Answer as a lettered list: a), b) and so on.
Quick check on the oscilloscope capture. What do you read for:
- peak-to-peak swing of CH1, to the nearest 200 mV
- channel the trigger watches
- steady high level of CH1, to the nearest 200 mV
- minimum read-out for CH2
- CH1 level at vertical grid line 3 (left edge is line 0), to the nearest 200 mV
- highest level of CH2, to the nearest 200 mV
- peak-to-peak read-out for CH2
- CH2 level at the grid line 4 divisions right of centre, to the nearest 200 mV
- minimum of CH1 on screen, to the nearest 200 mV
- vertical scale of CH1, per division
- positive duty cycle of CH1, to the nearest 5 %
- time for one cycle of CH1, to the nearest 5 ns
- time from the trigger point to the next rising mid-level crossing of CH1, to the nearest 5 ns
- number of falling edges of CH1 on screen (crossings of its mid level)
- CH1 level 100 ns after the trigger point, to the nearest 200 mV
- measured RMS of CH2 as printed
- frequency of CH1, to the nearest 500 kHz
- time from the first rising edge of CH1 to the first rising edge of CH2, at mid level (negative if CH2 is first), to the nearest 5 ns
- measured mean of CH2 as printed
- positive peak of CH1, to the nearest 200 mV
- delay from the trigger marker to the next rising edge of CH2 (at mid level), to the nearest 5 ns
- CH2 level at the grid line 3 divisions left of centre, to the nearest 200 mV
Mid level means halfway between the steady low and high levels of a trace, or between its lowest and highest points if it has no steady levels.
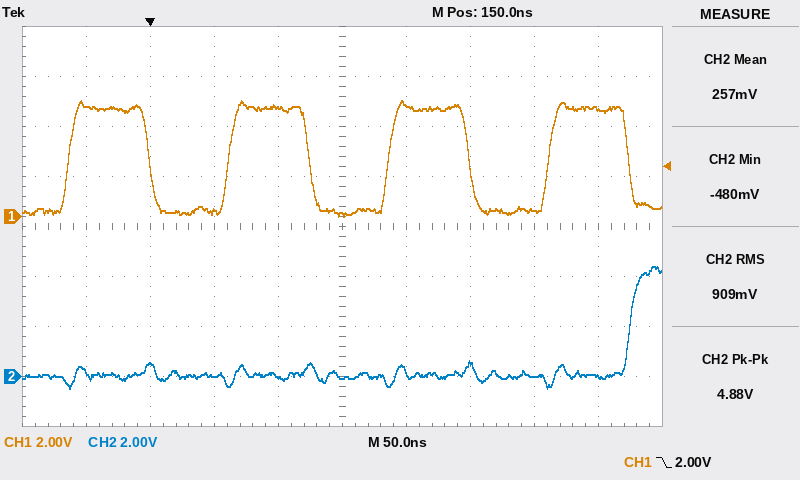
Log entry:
a) 4.6 V
b) CH1
c) 4.4 V
d) -480 mV
e) 200 mV
f) 4.4 V
g) 4.88 V
h) 0.0 V
i) 0.0 V
j) 2 V
k) 50 %
l) 125 ns
m) 60 ns
n) 4
o) 4.4 V
p) 909 mV
q) 8.0 MHz
r) +440 ns
s) 257 mV
t) 4.6 V
u) 375 ns
v) 600 mV
